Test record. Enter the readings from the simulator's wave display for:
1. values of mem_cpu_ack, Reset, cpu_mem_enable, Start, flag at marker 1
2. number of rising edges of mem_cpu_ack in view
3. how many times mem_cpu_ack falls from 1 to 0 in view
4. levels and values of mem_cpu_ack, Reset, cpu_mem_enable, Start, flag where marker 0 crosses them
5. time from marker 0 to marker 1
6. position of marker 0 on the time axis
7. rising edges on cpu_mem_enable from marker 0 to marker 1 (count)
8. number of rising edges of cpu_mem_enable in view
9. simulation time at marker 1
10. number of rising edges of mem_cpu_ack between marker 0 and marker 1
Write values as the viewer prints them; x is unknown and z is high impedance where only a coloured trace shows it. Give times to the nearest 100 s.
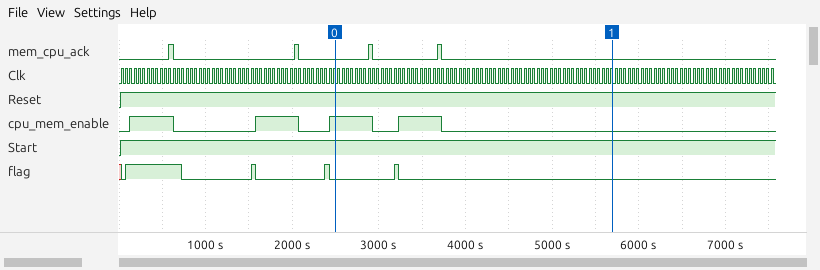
mem_cpu_ack=0, Reset=1, cpu_mem_enable=0, Start=1, flag=0
4
4
mem_cpu_ack=0, Reset=1, cpu_mem_enable=1, Start=1, flag=0
3200 s
2500 s
1
4
5700 s
2
